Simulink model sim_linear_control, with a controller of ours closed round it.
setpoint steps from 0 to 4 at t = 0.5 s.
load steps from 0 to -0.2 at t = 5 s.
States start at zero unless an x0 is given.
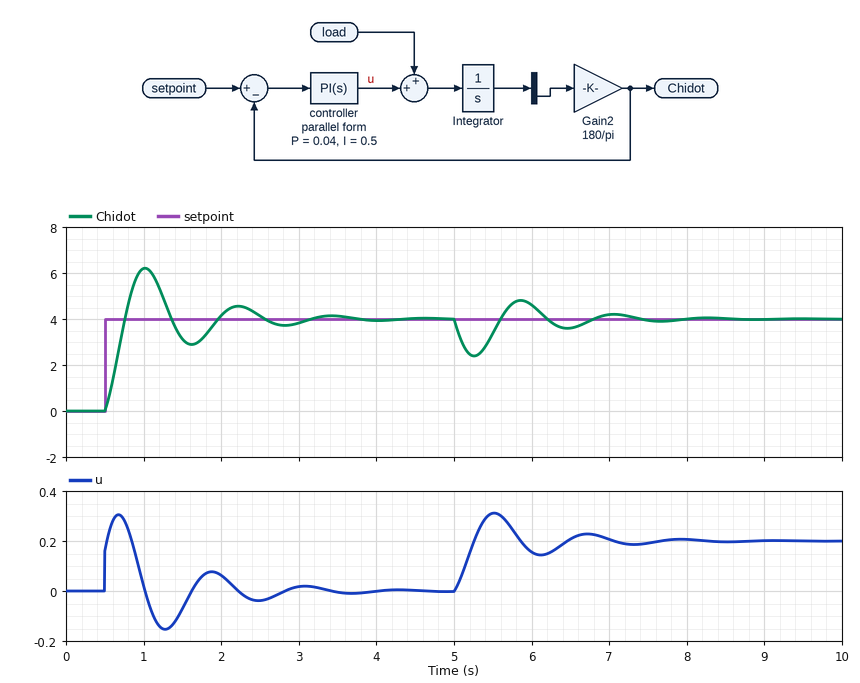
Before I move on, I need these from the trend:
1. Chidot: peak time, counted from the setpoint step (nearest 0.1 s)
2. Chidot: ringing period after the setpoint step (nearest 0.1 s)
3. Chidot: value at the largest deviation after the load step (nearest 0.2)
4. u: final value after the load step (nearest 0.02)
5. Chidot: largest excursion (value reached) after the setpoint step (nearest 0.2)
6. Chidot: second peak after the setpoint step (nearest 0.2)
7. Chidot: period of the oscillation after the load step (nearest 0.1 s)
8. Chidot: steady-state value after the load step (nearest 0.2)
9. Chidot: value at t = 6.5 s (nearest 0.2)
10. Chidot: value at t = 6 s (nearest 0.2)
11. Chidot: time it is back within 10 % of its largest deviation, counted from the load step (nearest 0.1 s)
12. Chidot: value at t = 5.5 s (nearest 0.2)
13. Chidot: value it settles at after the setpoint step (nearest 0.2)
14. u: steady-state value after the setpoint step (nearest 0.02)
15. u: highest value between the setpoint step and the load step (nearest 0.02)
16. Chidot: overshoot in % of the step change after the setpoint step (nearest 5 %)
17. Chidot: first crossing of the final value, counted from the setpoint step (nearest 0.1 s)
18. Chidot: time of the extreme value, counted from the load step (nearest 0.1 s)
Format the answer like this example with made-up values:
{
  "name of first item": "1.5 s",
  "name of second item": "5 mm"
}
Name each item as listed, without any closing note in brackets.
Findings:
{
  "Chidot: peak time, counted from the setpoint step": "0.5 s",
  "Chidot: ringing period after the setpoint step": "1.2 s",
  "Chidot: value at the largest deviation after the load step": "2.4",
  "u: final value after the load step": "0.20",
  "Chidot: largest excursion (value reached) after the setpoint step": "6.2",
  "Chidot: second peak after the setpoint step": "4.6",
  "Chidot: period of the oscillation after the load step": "1.2 s",
  "Chidot: steady-state value after the load step": "4.0",
  "Chidot: value at t = 6.5 s": "3.6",
  "Chidot: value at t = 6 s": "4.6",
  "Chidot: time it is back within 10 % of its largest deviation, counted from the load step": "2.2 s",
  "Chidot: value at t = 5.5 s": "3.4",
  "Chidot: value it settles at after the setpoint step": "4.0",
  "u: steady-state value after the setpoint step": "0.00",
  "u: highest value between the setpoint step and the load step": "0.30",
  "Chidot: overshoot in % of the step change after the setpoint step": "55 %",
  "Chidot: first crossing of the final value, counted from the setpoint step": "0.3 s",
  "Chidot: time of the extreme value, counted from the load step": "0.3 s"
}
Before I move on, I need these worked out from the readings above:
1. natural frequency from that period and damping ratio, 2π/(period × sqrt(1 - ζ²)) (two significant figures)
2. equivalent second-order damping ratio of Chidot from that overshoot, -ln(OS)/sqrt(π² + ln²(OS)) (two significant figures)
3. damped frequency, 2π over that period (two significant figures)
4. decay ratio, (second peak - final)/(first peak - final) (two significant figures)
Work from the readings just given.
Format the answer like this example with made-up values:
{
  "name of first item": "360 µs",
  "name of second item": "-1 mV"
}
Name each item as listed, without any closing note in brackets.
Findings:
{
  "natural frequency from that period and damping ratio, 2π/(period × sqrt(1 - ζ²))": "5.3 rad/s",
  "equivalent second-order damping ratio of Chidot from that overshoot, -ln(OS)/sqrt(π² + ln²(OS))": "0.19",
  "damped frequency, 2π over that period": "5.2 rad/s",
  "decay ratio, (second peak - final)/(first peak - final)": "0.27"
}
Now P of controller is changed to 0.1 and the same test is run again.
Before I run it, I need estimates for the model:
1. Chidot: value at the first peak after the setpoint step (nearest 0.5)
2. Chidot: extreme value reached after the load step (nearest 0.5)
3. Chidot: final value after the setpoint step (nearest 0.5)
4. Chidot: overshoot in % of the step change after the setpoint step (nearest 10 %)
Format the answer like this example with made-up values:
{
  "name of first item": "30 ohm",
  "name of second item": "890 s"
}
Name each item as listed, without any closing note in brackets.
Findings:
{
  "Chidot: value at the first peak after the setpoint step": "5.0",
  "Chidot: extreme value reached after the load step": "3.0",
  "Chidot: final value after the setpoint step": "4.0",
  "Chidot: overshoot in % of the step change after the setpoint step": "30 %"
}
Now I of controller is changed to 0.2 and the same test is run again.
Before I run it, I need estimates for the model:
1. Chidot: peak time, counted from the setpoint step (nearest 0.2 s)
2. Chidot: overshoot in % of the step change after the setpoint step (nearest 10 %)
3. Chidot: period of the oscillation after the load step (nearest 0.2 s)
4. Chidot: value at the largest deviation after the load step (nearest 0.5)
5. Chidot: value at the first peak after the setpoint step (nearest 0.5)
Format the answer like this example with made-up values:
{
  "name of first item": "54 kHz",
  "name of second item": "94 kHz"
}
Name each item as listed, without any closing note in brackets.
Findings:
{
  "Chidot: peak time, counted from the setpoint step": "0.8 s",
  "Chidot: overshoot in % of the step change after the setpoint step": "40 %",
  "Chidot: period of the oscillation after the load step": "2.0 s",
  "Chidot: value at the largest deviation after the load step": "2.0",
  "Chidot: value at the first peak after the setpoint step": "5.5"
}
